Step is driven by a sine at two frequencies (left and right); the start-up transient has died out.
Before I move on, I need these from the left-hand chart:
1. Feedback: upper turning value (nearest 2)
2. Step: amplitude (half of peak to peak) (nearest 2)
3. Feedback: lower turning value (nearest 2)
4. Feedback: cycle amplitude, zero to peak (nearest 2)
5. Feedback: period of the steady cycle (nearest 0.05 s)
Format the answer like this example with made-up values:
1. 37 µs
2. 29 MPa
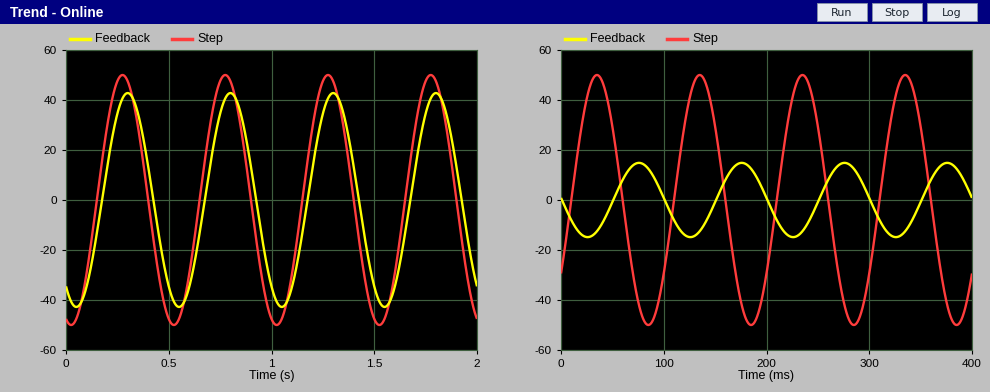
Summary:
1. 42
2. 50
3. -42
4. 42
5. 0.50 s
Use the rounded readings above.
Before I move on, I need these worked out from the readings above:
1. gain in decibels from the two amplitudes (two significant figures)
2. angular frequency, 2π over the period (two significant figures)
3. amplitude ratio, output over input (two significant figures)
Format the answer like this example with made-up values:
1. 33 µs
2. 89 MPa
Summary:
1. -1.5 dB
2. 13 rad/s
3. 0.84
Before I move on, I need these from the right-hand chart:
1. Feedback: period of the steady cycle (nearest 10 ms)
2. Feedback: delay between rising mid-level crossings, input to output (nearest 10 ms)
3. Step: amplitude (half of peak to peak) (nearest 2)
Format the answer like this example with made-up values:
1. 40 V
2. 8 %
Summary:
1. 100 ms
2. 40 ms
3. 50
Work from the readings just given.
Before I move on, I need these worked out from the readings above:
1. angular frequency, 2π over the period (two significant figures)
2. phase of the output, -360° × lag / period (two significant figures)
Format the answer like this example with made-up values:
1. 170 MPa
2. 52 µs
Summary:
1. 0.063 rad/ms
2. -140°
